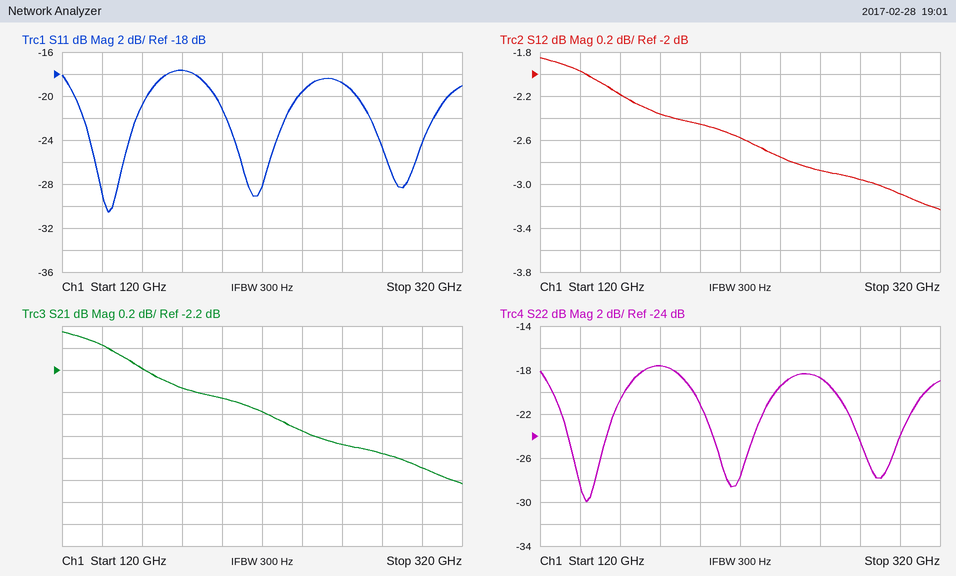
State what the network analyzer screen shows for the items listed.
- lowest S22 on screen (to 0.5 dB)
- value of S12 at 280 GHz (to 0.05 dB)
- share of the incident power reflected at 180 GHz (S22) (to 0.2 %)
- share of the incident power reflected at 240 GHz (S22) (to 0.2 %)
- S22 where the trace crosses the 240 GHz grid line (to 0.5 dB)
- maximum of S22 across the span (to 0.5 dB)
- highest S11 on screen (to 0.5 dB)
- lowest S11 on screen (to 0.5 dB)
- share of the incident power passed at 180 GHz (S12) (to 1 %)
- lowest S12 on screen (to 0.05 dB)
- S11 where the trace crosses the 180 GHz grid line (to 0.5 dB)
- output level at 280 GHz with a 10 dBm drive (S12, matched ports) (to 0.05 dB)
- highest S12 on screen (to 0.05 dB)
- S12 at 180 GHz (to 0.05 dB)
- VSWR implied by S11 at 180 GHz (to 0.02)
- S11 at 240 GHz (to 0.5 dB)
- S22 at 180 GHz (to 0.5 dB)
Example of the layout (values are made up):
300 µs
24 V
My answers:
-30.0 dB
-2.95 dB
1.8 %
1.2 %
-19.5 dB
-17.5 dB
-17.5 dB
-30.5 dB
58 %
-3.25 dB
-17.5 dB
7.05 dBm
-1.85 dB
-2.35 dB
1.30
-19.5 dB
-17.5 dB
